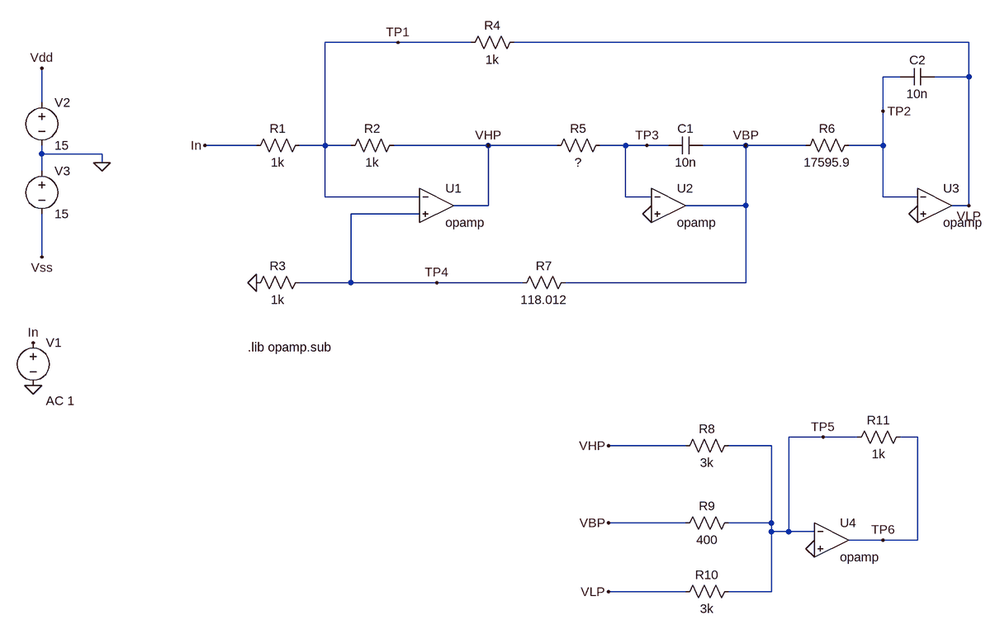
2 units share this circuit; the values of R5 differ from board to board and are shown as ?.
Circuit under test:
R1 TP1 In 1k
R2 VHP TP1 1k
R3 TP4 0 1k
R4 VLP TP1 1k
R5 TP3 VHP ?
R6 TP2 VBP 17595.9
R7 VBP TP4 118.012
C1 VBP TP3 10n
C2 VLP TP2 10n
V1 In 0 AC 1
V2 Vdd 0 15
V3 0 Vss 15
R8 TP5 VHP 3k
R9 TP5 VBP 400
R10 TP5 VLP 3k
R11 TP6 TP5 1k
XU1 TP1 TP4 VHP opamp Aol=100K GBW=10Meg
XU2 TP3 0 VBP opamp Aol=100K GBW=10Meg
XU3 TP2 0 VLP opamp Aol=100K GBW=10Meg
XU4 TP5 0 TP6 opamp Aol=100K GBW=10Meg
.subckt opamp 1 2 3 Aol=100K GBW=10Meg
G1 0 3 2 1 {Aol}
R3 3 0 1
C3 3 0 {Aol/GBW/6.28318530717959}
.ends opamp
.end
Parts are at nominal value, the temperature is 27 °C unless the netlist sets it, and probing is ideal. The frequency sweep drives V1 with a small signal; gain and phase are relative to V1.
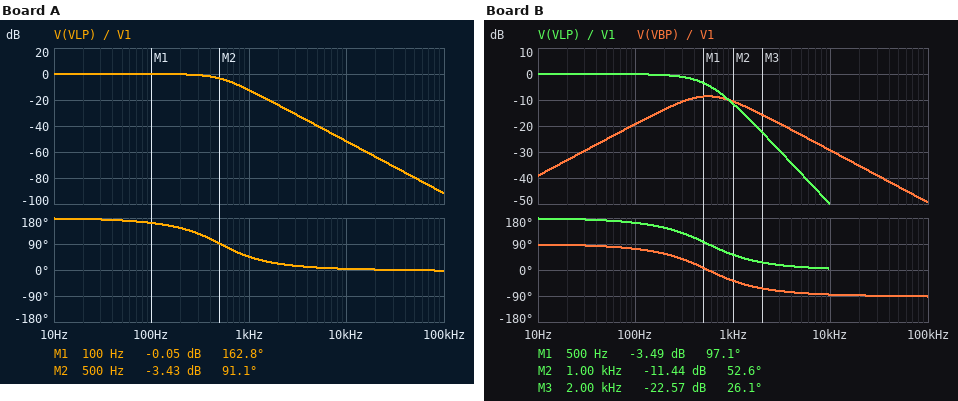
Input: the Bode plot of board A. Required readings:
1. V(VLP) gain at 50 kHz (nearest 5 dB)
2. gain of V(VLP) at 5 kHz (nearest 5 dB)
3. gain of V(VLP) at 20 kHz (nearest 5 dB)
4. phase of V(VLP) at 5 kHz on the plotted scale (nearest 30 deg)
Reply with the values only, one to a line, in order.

-80 dB
-40 dB
-65 dB
0 deg
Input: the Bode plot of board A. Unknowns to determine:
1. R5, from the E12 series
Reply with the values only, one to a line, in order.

56 kΩ
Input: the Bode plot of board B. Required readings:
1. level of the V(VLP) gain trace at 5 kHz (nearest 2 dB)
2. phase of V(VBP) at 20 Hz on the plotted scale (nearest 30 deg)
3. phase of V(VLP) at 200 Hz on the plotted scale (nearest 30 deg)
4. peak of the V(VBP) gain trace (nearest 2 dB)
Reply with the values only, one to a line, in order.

-38 dB
90 deg
150 deg
-8 dB
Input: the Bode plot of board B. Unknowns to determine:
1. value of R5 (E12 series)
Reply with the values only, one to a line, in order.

47 kΩ
